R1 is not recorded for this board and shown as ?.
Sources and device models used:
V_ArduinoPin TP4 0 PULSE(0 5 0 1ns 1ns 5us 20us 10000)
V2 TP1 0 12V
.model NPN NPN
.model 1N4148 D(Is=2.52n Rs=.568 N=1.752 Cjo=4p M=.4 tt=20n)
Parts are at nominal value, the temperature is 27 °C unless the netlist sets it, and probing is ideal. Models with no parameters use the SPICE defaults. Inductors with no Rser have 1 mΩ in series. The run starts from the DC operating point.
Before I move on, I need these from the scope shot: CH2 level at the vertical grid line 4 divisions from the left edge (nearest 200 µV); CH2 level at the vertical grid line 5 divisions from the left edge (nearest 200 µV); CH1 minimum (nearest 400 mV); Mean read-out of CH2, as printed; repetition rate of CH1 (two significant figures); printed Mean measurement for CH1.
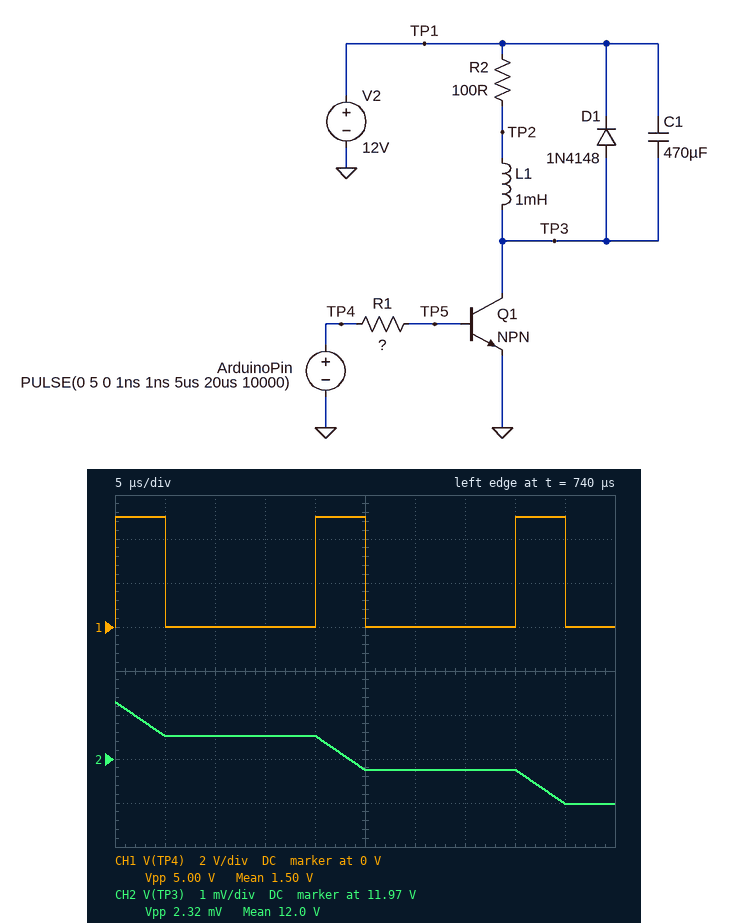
11.9706 V
11.9698 V
0 V
12.0 V
50 kHz
1.50 V
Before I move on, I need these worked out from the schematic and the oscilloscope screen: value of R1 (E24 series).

5.6 kΩ
